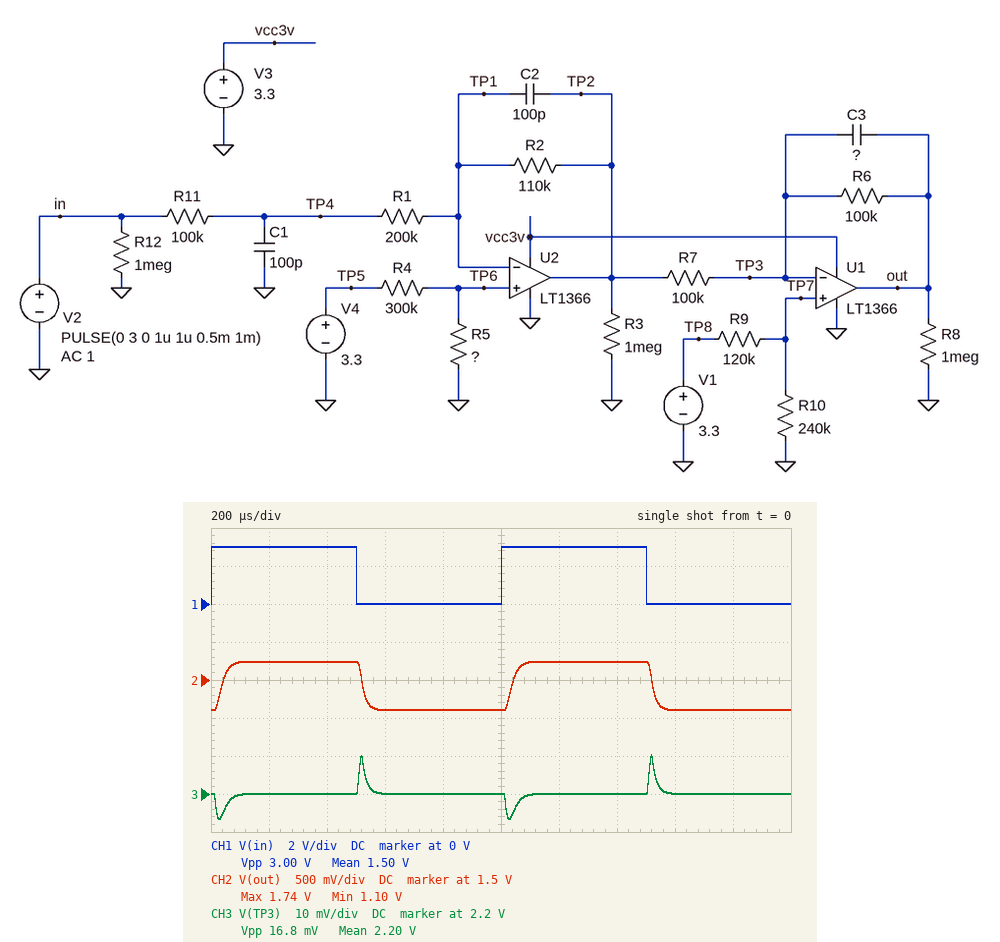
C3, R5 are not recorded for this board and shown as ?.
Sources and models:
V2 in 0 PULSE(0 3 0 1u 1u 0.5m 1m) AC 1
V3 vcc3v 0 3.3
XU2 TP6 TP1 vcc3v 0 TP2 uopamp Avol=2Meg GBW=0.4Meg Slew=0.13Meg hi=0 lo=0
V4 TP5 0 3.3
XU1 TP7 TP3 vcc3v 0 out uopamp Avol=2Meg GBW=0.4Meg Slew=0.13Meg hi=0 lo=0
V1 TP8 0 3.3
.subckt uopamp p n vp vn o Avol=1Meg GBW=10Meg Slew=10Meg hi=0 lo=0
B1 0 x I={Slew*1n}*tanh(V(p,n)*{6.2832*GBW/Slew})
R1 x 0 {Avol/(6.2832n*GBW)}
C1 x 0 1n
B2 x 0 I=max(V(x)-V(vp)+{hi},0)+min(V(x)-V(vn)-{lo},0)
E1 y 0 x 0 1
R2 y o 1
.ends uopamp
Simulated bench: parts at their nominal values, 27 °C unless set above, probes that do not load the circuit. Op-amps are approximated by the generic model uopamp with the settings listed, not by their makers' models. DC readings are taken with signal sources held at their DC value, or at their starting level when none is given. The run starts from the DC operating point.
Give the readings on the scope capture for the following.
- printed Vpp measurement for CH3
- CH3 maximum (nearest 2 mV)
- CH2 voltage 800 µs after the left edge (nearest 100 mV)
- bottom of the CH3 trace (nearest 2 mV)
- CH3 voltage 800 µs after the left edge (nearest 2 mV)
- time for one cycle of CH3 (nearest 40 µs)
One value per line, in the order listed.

16.8 mV
2.210 V
1.1 V
2.194 V
2.200 V
1.00 ms
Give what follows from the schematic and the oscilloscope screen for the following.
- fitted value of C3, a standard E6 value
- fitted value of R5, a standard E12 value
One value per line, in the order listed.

150 pF
1.5 MΩ
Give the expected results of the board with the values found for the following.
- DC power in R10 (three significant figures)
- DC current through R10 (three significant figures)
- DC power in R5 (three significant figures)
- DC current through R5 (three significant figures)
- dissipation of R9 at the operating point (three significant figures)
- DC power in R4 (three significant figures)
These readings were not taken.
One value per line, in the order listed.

20.2 µW
9.17 µA
5.04 µW
1.83 µA
10.1 µW
1.01 µW
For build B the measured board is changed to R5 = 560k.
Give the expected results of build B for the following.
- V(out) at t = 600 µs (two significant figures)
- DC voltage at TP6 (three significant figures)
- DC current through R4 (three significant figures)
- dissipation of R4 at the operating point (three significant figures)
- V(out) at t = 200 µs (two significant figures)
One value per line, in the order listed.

1.5 V
2.15 V
3.84 µA
4.42 µW
2.6 V
